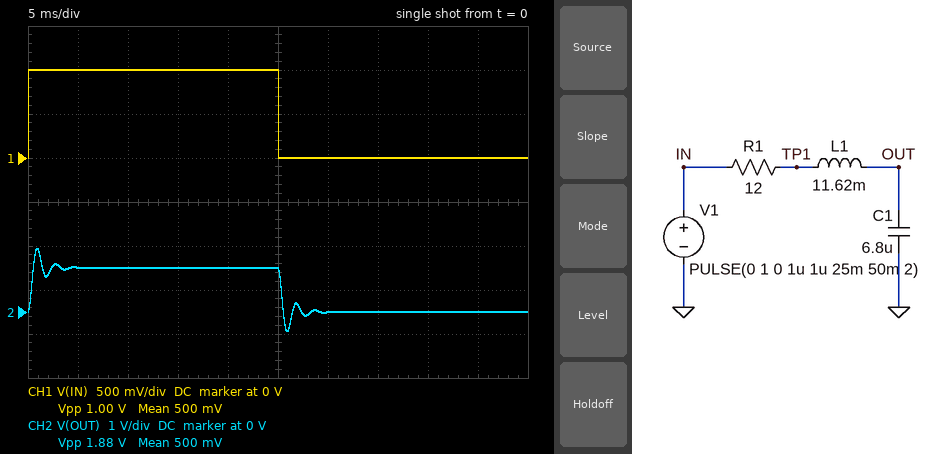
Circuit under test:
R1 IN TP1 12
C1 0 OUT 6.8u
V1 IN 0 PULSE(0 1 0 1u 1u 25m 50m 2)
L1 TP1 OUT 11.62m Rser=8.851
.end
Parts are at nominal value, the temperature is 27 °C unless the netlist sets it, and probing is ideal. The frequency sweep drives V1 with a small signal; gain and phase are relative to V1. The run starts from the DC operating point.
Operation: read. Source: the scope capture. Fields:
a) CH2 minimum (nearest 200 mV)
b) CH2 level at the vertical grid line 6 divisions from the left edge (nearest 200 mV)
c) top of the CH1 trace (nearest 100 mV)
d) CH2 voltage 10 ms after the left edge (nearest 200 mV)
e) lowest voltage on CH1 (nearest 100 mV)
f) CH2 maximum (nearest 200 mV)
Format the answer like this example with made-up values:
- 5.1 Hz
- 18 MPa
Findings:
- -400 mV
- 0 V
- 1.0 V
- 1.0 V
- 0 V
- 1.4 V
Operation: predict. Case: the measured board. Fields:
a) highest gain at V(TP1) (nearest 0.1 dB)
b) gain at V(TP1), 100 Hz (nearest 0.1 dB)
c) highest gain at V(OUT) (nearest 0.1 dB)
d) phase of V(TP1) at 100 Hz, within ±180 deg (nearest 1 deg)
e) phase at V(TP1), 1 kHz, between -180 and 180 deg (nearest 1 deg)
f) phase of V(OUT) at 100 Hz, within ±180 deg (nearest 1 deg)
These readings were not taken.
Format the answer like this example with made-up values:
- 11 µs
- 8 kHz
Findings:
- 0 dB
- 0 dB
- 6.2 dB
- -3 deg
- 13 deg
- -5 deg
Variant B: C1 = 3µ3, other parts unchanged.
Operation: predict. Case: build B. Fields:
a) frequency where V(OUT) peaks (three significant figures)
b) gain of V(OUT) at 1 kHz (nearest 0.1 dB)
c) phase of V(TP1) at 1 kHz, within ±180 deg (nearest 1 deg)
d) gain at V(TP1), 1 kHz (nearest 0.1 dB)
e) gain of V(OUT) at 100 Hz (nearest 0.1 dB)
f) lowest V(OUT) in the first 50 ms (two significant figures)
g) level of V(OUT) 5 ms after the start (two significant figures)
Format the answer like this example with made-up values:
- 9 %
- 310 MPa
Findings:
- 787 Hz
- 3.5 dB
- 20 deg
- -1.8 dB
- 0.1 dB
- -570 mV
- 990 mV
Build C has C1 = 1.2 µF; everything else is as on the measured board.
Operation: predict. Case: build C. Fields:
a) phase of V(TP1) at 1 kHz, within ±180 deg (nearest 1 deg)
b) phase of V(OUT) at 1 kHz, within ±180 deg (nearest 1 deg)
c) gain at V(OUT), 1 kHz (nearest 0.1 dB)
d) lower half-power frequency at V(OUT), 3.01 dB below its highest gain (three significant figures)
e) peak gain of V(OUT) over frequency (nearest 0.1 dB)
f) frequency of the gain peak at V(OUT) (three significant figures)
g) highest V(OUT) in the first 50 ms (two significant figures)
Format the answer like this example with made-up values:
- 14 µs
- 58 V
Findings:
- -11 deg
- -19 deg
- 6.4 dB
- 1.18 kHz
- 13.5 dB
- 1.33 kHz
- 1.7 V
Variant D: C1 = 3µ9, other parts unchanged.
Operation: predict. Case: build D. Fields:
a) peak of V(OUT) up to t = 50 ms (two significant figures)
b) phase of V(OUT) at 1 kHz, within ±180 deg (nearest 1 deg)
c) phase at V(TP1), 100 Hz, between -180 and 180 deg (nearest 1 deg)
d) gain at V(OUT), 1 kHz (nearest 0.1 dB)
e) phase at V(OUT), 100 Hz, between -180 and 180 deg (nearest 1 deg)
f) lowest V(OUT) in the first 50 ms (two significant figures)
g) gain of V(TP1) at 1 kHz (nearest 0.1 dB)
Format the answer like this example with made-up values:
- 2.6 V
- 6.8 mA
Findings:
- 1.5 V
- -147 deg
- -2 deg
- 0.5 dB
- -3 deg
- -540 mV
- -1.2 dB
